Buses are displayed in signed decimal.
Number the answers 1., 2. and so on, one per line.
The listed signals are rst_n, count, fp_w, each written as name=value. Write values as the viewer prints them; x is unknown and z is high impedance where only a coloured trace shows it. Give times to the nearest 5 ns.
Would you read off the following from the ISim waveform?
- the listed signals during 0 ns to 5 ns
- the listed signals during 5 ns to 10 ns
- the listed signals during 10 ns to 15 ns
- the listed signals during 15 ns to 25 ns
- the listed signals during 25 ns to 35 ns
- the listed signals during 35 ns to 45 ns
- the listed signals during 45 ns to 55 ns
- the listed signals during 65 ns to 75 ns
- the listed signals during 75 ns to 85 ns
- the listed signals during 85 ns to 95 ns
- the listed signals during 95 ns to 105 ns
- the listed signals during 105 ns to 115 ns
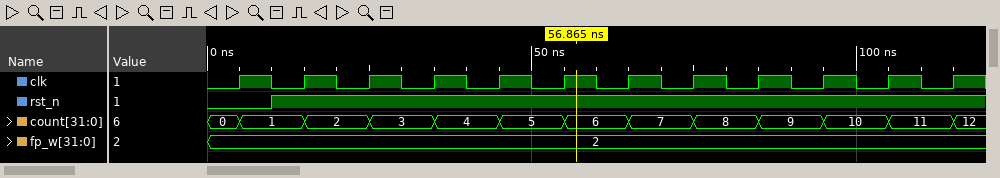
1. rst_n=0, count=0, fp_w=2
2. rst_n=0, count=1, fp_w=2
3. rst_n=1, count=1, fp_w=2
4. rst_n=1, count=2, fp_w=2
5. rst_n=1, count=3, fp_w=2
6. rst_n=1, count=4, fp_w=2
7. rst_n=1, count=5, fp_w=2
8. rst_n=1, count=7, fp_w=2
9. rst_n=1, count=8, fp_w=2
10. rst_n=1, count=9, fp_w=2
11. rst_n=1, count=10, fp_w=2
12. rst_n=1, count=11, fp_w=2
